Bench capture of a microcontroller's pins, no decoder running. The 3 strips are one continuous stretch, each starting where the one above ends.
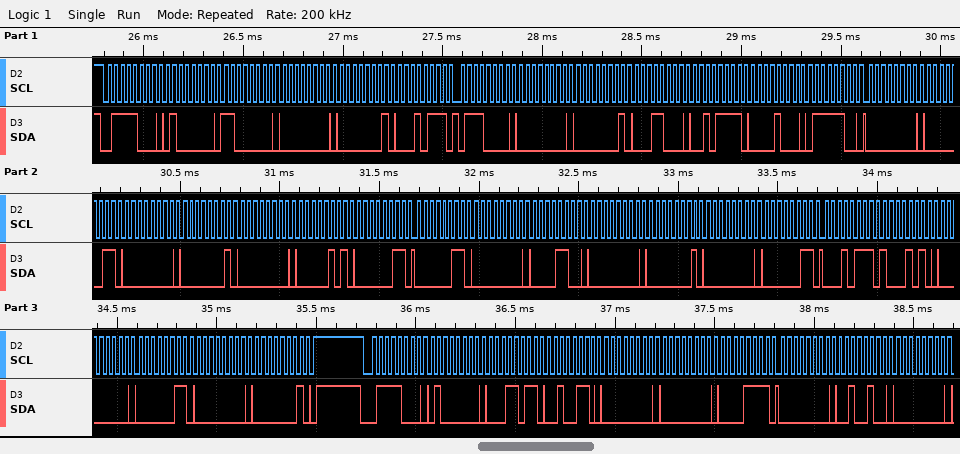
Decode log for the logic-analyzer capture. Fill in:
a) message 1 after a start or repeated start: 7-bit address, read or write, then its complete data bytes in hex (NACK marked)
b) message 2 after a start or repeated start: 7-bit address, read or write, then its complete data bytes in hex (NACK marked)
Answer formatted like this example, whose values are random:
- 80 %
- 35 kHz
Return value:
- 0x3C write: 40 C0 00 01 17 70 00 01 18 2F 08 7C 00 03 00 01 00 05 03 03 00 0C 00 01 00 03 17 8A 00 03 00 01
- 0x3C write: 40 1B 26 00 00 0F 00 24 00
